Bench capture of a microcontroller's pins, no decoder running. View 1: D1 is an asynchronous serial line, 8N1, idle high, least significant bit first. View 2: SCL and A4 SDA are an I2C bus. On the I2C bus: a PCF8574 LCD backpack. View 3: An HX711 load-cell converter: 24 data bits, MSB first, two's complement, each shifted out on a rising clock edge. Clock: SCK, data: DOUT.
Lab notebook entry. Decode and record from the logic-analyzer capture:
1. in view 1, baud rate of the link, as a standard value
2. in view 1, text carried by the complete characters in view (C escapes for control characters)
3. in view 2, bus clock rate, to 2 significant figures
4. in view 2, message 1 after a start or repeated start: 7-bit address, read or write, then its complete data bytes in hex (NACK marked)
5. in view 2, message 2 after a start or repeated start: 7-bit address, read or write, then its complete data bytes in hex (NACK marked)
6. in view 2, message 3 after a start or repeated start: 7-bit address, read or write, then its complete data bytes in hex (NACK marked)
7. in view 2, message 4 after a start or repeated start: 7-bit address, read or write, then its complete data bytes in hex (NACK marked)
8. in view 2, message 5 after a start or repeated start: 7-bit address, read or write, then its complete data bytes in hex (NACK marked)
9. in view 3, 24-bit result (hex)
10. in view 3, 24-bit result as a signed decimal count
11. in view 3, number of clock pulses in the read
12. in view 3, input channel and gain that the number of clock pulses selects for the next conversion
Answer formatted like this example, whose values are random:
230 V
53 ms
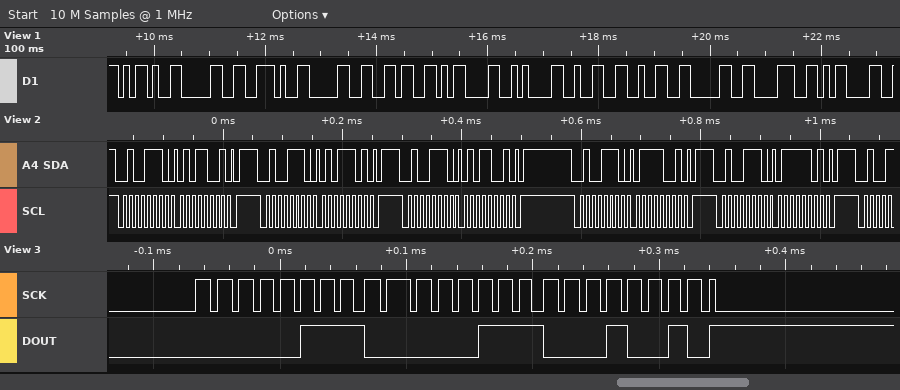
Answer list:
9600 baud
"-0.06\r\n2208\r"
100 kHz
0x27 write: 59
0x27 write: 5D
0x27 write: 59
0x27 write: 79
0x27 write: 7D
0x070712
460562
25
channel A, gain 128
